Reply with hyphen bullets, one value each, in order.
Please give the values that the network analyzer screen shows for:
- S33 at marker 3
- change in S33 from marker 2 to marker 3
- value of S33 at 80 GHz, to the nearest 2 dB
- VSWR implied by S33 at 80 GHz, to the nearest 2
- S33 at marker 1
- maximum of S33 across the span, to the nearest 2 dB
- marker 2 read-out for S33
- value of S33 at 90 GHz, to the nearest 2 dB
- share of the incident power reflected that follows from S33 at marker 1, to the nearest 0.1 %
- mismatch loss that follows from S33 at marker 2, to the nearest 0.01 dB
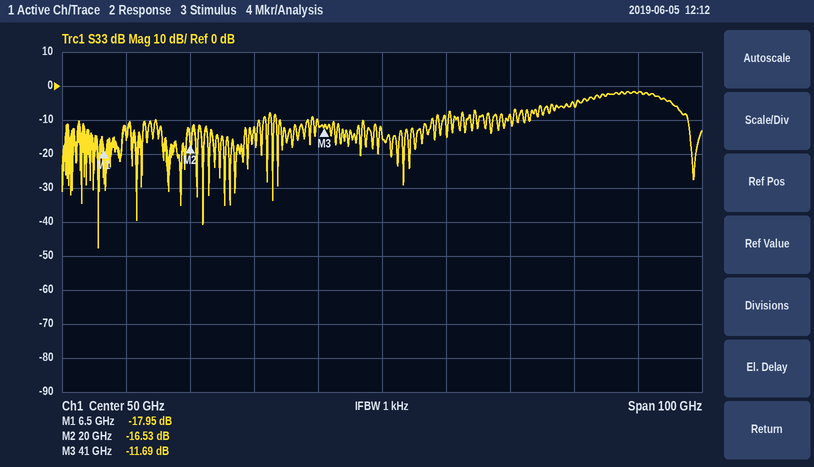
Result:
- -11.69 dB
- 4.84 dB
- -6 dB
- 4
- -17.95 dB
- -2 dB
- -16.53 dB
- -2 dB
- 1.6 %
- 0.10 dB
